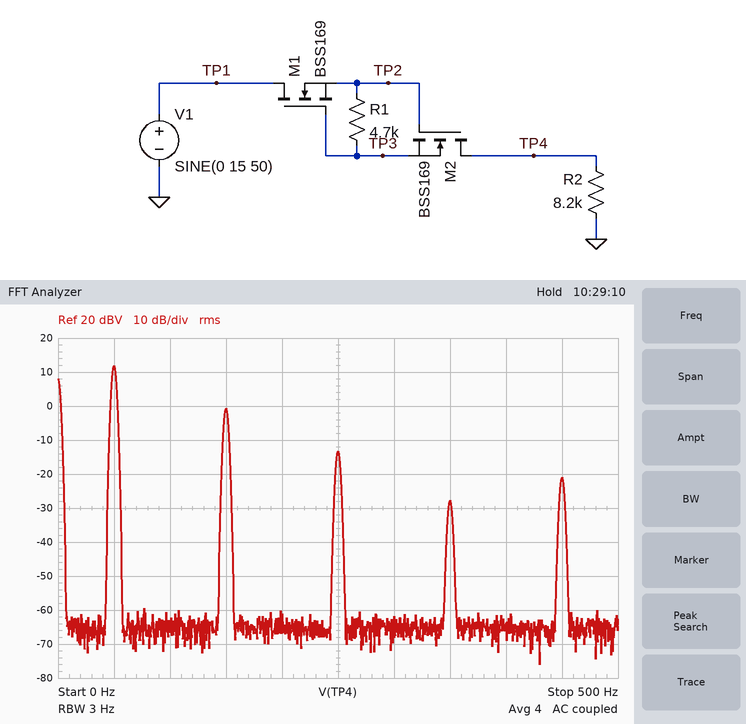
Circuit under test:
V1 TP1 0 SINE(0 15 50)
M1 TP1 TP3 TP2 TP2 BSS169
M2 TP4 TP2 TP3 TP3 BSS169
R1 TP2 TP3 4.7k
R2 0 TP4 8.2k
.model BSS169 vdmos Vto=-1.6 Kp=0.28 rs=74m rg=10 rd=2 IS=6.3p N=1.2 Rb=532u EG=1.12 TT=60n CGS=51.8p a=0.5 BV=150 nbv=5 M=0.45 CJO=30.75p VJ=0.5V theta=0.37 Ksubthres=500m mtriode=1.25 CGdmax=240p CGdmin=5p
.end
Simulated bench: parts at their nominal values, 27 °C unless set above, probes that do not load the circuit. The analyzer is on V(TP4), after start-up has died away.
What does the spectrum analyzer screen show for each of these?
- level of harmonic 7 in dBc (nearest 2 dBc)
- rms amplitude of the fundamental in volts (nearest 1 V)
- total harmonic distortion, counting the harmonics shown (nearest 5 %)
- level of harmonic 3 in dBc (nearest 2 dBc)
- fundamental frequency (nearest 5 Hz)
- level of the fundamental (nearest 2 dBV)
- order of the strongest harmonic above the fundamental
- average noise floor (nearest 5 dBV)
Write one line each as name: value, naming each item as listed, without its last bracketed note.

level of harmonic 7 in dBc: -40 dBc
rms amplitude of the fundamental in volts: 4 V
total harmonic distortion, counting the harmonics shown: 25 %
level of harmonic 3 in dBc: -12 dBc
fundamental frequency: 50 Hz
level of the fundamental: 12 dBV
order of the strongest harmonic above the fundamental: 3
average noise floor: -65 dBV
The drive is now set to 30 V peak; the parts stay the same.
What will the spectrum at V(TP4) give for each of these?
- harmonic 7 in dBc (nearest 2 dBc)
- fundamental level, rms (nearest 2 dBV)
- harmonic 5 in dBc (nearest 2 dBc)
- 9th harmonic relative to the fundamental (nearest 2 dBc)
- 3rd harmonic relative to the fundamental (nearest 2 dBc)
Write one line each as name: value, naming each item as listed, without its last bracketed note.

harmonic 7 in dBc: -22 dBc
fundamental level, rms: 12 dBV
harmonic 5 in dBc: -16 dBc
9th harmonic relative to the fundamental: -28 dBc
3rd harmonic relative to the fundamental: -10 dBc
